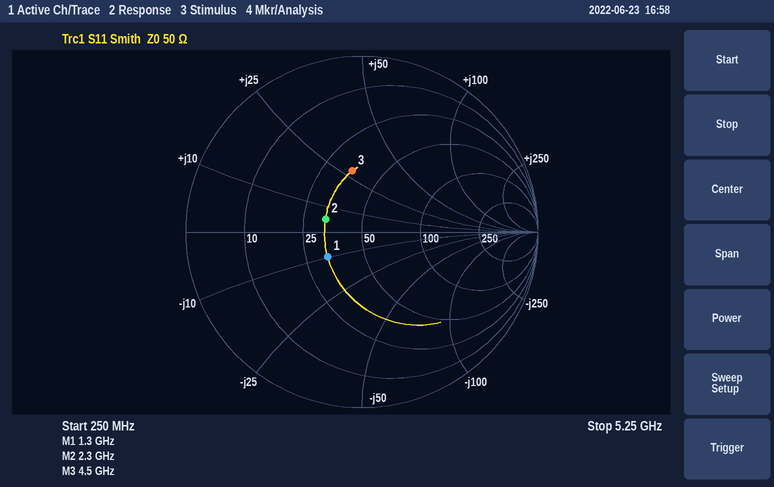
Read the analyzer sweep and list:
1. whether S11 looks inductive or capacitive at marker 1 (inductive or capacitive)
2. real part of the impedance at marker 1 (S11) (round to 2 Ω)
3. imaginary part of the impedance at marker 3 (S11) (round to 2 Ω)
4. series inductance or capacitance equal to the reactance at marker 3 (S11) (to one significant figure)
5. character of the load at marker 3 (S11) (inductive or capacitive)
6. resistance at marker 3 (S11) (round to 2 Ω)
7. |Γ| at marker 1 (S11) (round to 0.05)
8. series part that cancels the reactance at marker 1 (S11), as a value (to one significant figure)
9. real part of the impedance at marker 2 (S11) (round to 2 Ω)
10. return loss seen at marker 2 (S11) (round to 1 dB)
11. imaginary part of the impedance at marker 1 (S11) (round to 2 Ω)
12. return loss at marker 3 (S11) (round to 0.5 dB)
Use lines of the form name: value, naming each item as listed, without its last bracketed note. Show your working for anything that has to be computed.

whether S11 looks inductive or capacitive at marker 1: capacitive
real part of the impedance at marker 1 (S11): 32 Ω
imaginary part of the impedance at marker 3 (S11): +28 Ω
series inductance or capacitance equal to the reactance at marker 3 (S11): L = 28 Ω/(2π × 4.5 GHz) ≈ 1.0 nH
character of the load at marker 3 (S11): inductive
resistance at marker 3 (S11): 36 Ω
|Γ| at marker 1 (S11): 0.25
series part that cancels the reactance at marker 1 (S11), as a value: L = 10 Ω/(2π × 1.3 GHz) ≈ 1 nH
real part of the impedance at marker 2 (S11): 32 Ω
return loss seen at marker 2 (S11): 13 dB
imaginary part of the impedance at marker 1 (S11): -10 Ω
return loss at marker 3 (S11): 9.0 dB
